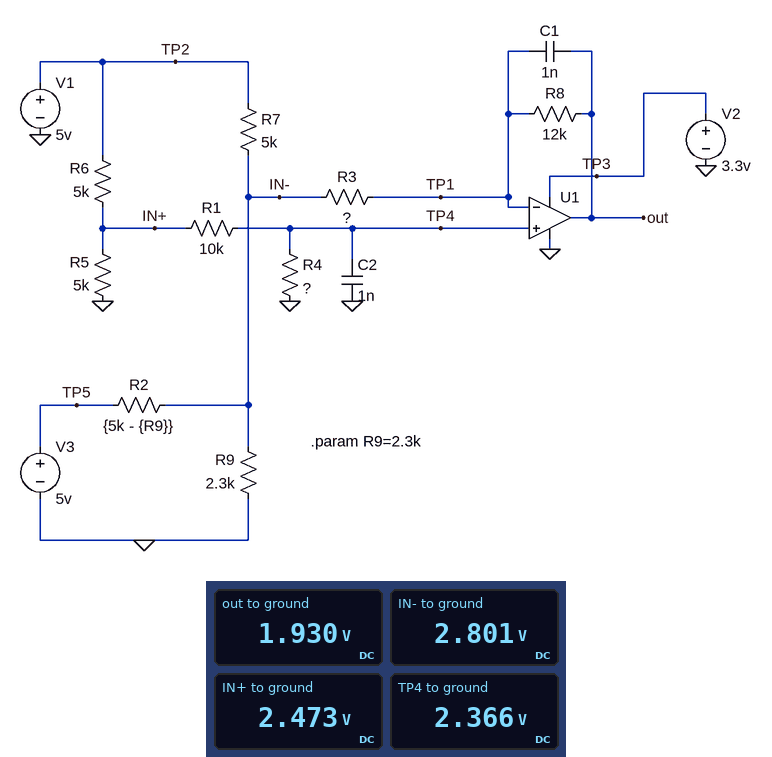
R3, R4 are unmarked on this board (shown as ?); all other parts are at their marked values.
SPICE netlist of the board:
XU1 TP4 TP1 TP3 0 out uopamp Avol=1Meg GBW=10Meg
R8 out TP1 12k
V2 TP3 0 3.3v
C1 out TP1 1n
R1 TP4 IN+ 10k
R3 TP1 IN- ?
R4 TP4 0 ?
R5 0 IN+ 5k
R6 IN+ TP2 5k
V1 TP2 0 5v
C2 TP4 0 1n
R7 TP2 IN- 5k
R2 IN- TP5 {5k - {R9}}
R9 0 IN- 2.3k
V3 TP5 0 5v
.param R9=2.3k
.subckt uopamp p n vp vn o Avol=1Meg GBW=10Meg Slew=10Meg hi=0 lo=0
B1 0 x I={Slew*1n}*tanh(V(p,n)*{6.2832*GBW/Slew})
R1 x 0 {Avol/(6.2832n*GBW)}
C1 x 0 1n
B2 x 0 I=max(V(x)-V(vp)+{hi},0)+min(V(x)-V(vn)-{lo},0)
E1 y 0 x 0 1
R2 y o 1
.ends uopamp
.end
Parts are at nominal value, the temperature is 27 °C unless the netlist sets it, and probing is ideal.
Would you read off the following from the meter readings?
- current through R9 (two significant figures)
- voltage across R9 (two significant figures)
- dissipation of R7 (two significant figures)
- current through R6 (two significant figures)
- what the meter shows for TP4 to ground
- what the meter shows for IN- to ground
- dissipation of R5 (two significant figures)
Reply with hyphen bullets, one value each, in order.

- 1.2 mA
- 2.8 V
- 970 µW
- 510 µA
- 2.366 V
- 2.801 V
- 1.2 mW
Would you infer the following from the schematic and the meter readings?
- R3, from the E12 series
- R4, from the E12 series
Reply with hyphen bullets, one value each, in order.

- 12 kΩ
- 220 kΩ
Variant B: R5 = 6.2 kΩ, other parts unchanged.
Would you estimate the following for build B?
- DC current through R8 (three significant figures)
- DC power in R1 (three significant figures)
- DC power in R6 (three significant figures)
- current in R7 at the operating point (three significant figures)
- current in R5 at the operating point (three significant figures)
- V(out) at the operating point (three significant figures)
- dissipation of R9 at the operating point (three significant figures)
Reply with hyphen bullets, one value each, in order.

- 17.0 µA
- 1.41 µW
- 1.03 mW
- 436 µA
- 441 µA
- 2.41 V
- 3.46 mW
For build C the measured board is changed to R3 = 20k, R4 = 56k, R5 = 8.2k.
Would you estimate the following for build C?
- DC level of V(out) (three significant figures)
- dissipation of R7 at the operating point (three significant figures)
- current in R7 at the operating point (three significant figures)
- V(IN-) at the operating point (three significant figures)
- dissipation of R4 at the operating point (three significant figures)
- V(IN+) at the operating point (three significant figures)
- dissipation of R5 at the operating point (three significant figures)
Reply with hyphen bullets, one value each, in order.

- 2.33 V
- 949 µW
- 436 µA
- 2.82 V
- 113 µW
- 2.97 V
- 1.07 mW
